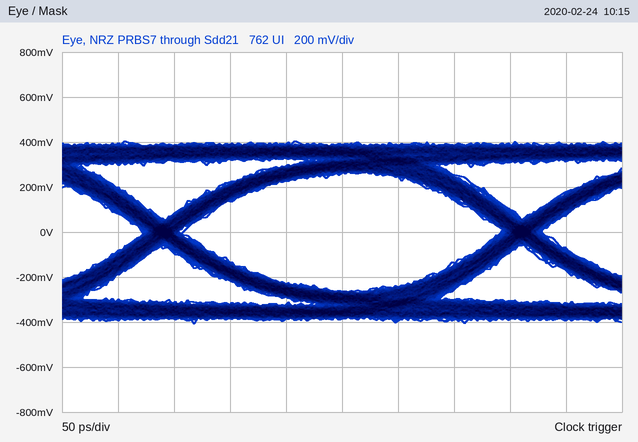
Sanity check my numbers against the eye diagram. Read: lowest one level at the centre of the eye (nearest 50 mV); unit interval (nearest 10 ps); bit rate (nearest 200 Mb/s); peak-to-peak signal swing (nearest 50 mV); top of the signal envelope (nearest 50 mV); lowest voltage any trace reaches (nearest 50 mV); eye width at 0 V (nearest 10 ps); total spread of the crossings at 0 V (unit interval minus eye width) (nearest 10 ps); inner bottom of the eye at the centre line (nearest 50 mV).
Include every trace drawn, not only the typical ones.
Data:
250 mV
320 ps
3.2 Gb/s
800 mV
400 mV
-400 mV
280 ps
40 ps
-250 mV
